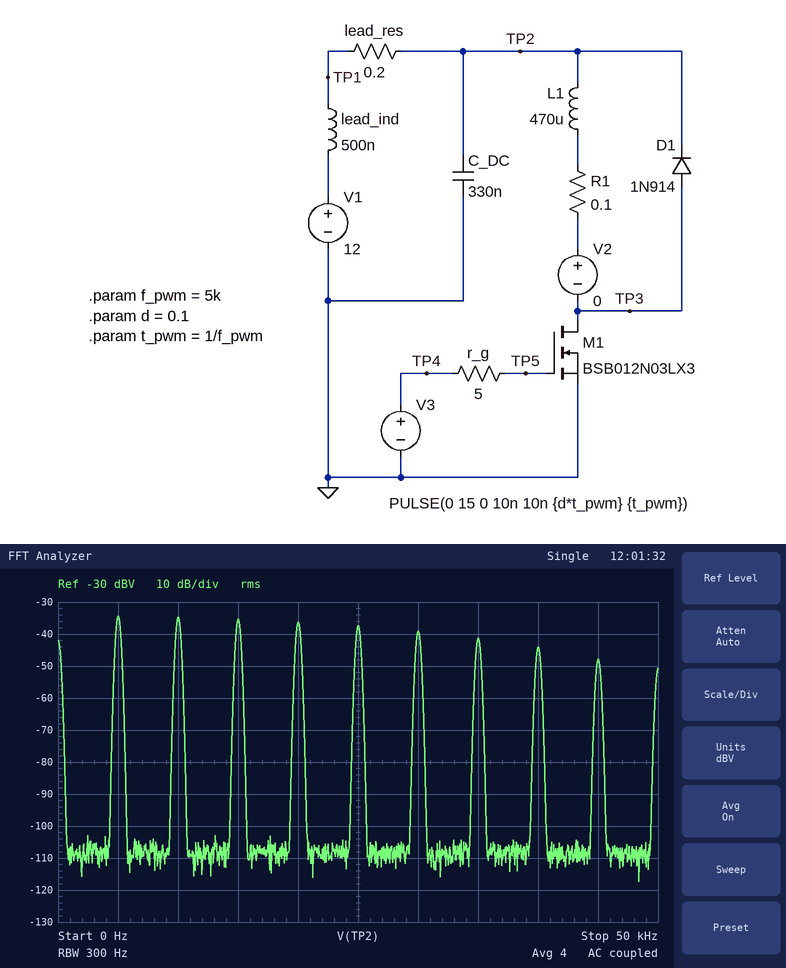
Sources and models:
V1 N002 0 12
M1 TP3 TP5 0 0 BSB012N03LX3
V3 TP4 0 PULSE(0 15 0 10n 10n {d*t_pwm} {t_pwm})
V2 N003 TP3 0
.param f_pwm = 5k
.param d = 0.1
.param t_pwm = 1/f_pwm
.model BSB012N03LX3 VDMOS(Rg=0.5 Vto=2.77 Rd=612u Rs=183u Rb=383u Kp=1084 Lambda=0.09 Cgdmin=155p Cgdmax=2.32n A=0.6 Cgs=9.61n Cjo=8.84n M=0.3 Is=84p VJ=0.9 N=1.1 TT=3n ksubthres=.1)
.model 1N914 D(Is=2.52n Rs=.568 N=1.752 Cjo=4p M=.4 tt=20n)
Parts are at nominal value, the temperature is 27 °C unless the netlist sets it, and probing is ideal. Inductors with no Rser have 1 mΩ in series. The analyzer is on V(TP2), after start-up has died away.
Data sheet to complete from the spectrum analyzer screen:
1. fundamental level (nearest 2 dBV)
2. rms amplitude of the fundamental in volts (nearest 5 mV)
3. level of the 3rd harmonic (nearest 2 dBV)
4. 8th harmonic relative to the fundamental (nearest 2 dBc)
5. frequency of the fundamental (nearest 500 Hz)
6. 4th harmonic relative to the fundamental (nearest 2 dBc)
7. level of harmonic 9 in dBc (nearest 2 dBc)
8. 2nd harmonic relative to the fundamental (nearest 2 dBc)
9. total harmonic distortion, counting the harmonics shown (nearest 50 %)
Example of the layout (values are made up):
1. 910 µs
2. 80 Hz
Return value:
1. -34 dBV
2. 20 mV
3. -36 dBV
4. -10 dBc
5. 5.0 kHz
6. -2 dBc
7. -14 dBc
8. 0 dBc
9. 200 %
